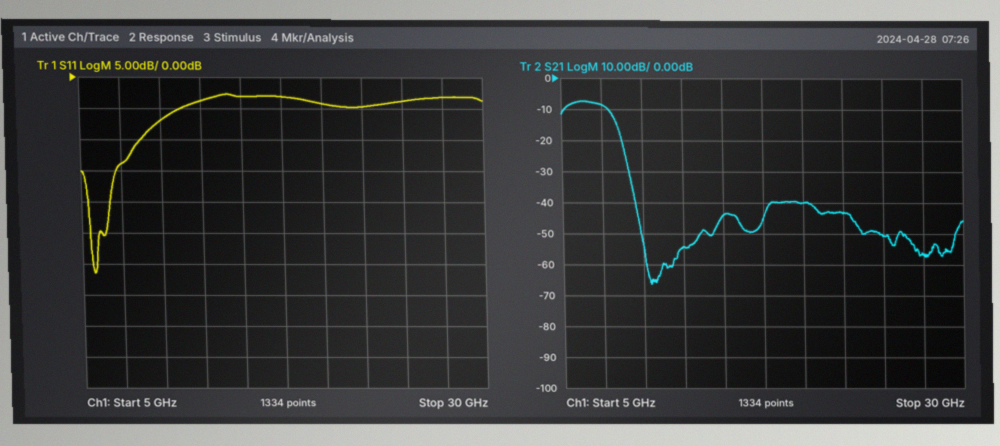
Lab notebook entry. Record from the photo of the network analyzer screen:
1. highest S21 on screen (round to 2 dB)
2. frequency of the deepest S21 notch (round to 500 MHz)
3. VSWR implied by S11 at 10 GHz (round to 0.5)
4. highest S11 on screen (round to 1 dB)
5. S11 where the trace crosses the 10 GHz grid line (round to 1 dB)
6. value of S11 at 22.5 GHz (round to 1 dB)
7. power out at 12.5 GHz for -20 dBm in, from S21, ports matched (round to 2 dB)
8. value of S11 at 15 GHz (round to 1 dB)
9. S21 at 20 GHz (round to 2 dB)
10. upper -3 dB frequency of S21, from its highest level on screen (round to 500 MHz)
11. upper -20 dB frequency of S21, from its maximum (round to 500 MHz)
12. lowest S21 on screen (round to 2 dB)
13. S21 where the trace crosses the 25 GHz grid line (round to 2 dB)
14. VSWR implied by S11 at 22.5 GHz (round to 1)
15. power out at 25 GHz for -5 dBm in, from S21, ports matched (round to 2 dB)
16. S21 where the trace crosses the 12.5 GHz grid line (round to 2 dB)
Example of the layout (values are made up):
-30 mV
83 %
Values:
-8 dB
10.5 GHz
2.5
-3 dB
-7 dB
-5 dB
-74 dBm
-3 dB
-40 dB
8.0 GHz
9.0 GHz
-66 dB
-50 dB
4
-56 dBm
-54 dB
